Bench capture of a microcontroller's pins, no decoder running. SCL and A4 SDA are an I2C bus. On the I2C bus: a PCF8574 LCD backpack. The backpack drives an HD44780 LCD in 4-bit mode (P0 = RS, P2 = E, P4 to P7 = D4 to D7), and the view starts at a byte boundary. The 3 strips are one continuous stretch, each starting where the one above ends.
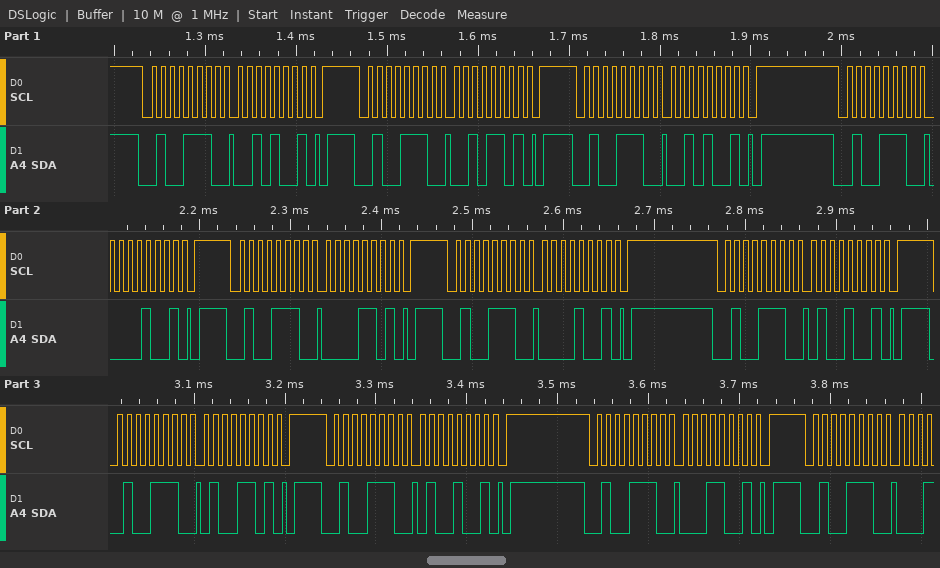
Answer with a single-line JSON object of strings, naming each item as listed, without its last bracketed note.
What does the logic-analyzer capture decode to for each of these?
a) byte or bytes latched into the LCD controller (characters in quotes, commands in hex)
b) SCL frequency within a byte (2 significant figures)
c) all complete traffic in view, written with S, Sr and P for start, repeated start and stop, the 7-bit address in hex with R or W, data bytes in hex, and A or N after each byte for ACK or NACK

{"byte or bytes latched into the LCD controller": "' '", "SCL frequency within a byte": "100 kHz", "all complete traffic in view, written with S, Sr and P for start, repeated start and stop, the 7-bit address in hex with R or W, data bytes in hex, and A or N after each byte for ACK or NACK": "S 27W A 29 A P S 27W A 2D A P S 27W A 29 A P S 27W A 09 A P S 27W A 0D A P S 27W A 09 A P S 27W A 49 A P S 27W A 4D A P S 27W A 49 A P S 27W A 19 A P S 27W A"}
